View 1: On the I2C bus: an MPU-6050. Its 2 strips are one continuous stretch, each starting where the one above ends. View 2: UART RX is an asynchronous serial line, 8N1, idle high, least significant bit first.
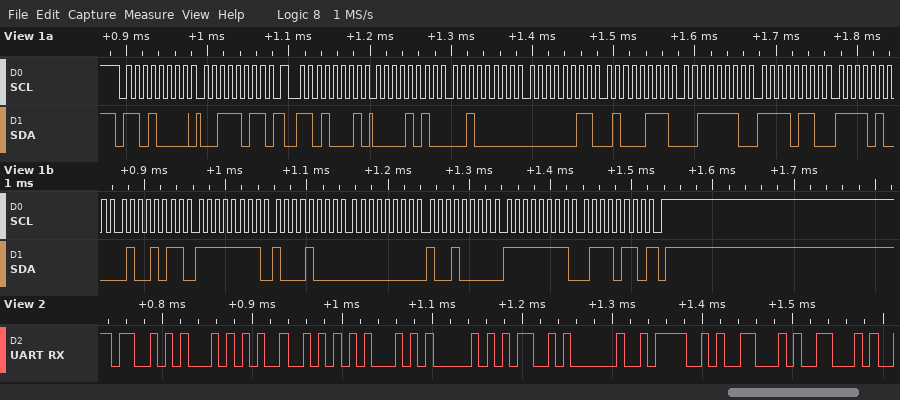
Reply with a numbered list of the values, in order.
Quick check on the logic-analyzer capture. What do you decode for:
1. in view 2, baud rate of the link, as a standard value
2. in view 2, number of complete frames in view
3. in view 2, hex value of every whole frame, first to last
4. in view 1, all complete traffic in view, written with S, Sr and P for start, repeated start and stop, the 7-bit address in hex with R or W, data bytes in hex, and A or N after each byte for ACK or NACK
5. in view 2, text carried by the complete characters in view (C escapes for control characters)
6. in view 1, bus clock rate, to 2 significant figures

1. 115200 baud
2. 10
3. 0x53 0x54 0x52 0x45 0x41 0x4D 0x20 0x4F 0x46 0x46
4. S 68W A 3B A Sr 68R A 0A A 20 A 03 A 47 A 3E A F6 A F4 A 4B A FF A 88 A 00 A 90 A FF A 76 N P
5. "STREAM OFF"
6. 100 kHz
